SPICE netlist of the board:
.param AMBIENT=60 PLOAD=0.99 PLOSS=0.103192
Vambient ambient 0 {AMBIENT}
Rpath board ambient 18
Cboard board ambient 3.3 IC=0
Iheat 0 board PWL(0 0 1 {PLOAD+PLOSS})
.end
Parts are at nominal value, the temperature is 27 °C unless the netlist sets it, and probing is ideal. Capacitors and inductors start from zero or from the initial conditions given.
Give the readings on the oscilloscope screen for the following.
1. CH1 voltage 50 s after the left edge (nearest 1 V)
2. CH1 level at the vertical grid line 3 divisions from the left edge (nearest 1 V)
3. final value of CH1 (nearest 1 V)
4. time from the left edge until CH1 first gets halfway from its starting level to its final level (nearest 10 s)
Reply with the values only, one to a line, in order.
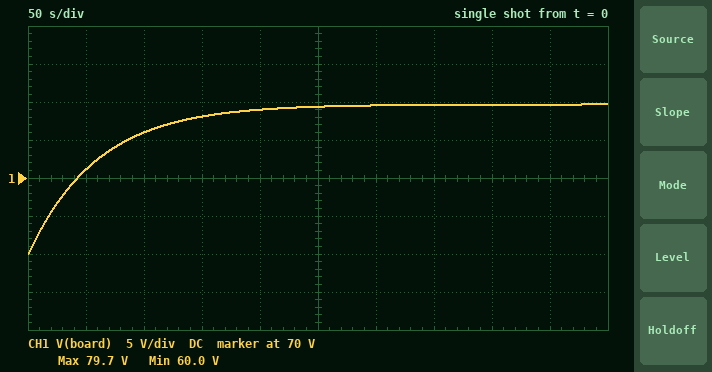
71 V
78 V
80 V
40 s
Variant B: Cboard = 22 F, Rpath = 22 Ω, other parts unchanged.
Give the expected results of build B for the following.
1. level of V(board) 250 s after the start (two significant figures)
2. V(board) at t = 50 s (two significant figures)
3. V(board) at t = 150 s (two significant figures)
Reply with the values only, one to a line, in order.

70 V
62 V
66 V
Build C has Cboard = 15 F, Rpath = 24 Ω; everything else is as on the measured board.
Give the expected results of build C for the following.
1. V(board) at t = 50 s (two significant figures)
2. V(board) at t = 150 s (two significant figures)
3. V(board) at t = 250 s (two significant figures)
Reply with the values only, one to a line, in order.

63 V
69 V
73 V
